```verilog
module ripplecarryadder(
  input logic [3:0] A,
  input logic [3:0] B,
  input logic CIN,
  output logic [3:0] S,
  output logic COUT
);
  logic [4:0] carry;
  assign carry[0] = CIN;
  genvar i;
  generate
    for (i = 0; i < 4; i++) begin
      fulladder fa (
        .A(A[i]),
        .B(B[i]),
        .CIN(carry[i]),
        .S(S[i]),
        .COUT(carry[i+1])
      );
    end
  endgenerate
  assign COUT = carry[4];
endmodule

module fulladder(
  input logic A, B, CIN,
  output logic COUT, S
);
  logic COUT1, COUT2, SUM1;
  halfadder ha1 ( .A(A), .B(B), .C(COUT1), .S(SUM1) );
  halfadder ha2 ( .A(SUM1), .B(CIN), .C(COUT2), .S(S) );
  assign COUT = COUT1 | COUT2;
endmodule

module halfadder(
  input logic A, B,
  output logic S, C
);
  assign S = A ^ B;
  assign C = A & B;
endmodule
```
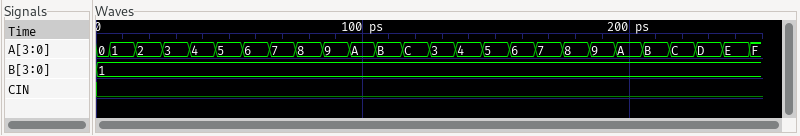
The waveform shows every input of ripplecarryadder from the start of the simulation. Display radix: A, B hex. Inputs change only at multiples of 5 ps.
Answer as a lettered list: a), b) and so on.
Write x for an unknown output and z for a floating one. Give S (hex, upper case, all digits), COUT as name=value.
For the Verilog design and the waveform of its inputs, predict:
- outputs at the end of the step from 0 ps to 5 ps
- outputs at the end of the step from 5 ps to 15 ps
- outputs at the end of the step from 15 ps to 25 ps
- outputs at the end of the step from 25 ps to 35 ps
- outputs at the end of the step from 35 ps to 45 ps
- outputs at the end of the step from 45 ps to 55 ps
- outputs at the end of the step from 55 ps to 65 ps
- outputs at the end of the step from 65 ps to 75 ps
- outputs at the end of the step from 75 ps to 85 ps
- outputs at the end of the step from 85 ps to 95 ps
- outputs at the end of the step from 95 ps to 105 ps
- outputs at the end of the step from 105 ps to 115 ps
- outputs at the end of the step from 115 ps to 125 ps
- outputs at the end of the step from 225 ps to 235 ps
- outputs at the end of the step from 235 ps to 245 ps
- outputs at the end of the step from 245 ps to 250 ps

a) S=1, COUT=0
b) S=2, COUT=0
c) S=3, COUT=0
d) S=4, COUT=0
e) S=5, COUT=0
f) S=6, COUT=0
g) S=7, COUT=0
h) S=8, COUT=0
i) S=9, COUT=0
j) S=A, COUT=0
k) S=B, COUT=0
l) S=C, COUT=0
m) S=D, COUT=0
n) S=E, COUT=0
o) S=F, COUT=0
p) S=0, COUT=1
